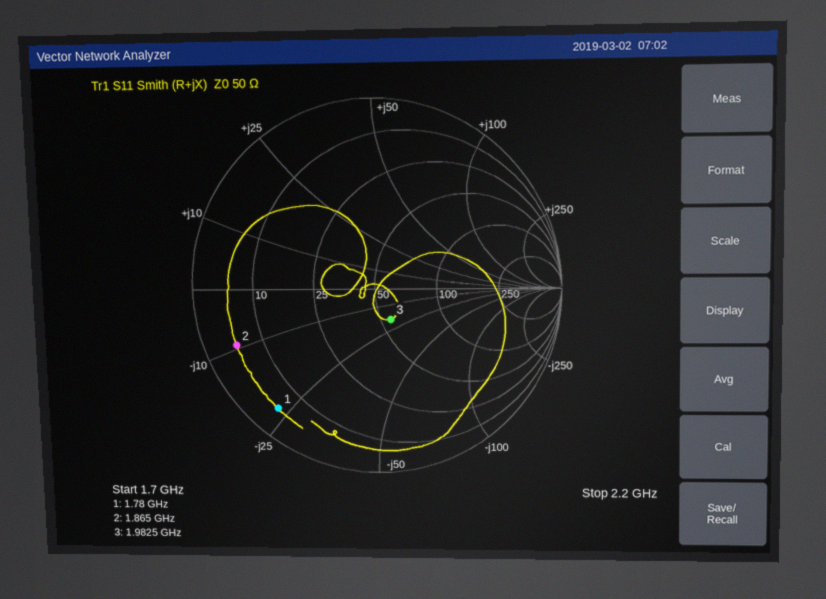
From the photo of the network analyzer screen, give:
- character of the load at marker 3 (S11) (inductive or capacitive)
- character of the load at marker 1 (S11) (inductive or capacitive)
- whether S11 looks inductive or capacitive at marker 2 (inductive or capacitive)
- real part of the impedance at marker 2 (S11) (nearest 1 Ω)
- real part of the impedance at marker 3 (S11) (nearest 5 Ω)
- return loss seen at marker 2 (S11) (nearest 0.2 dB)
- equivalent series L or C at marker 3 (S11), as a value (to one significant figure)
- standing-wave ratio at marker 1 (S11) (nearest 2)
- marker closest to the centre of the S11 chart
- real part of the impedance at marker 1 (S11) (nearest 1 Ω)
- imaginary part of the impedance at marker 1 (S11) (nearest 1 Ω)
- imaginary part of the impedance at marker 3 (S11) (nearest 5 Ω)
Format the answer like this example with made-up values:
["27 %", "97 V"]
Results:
["capacitive", "capacitive", "capacitive", "5 Ω", "55 Ω", "1.6 dB", "4 pF", "12", "marker 3", "5 Ω", "-23 Ω", "-20 Ω"]
